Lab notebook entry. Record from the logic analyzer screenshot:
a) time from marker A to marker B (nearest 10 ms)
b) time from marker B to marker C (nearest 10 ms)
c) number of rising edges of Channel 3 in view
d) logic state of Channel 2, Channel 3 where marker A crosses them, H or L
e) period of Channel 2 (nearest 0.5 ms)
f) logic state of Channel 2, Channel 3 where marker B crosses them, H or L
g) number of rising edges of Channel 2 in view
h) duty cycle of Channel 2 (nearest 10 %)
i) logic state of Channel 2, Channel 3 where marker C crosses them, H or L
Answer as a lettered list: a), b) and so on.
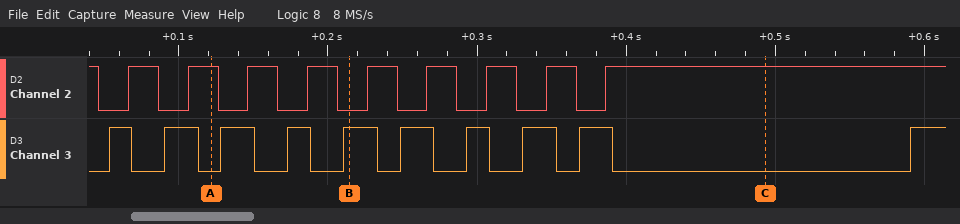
a) 90 ms
b) 280 ms
c) 10
d) Channel 2=H, Channel 3=L
e) 40 ms
f) Channel 2=L, Channel 3=H
g) 9
h) 50 %
i) Channel 2=H, Channel 3=L
